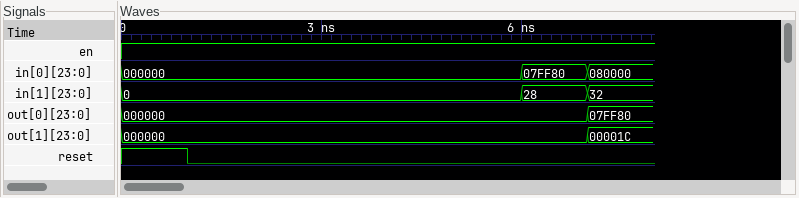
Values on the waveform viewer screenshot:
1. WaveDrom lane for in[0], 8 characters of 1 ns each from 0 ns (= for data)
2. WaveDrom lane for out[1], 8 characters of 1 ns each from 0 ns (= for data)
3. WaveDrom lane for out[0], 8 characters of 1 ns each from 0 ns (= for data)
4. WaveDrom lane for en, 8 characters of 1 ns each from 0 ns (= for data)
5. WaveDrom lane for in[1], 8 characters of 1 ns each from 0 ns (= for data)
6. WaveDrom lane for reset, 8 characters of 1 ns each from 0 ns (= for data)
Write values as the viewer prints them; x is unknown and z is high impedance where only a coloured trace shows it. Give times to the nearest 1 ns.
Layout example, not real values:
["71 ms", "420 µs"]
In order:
["{name: 'in[0]', wave: '=.....==', data: '000000 07FF80 080000'}", "{name: 'out[1]', wave: '=......=', data: '000000 00001C'}", "{name: 'out[0]', wave: '=......=', data: '000000 07FF80'}", "{name: 'en', wave: '1.......'}", "{name: 'in[1]', wave: '=.....==', data: '0 28 32'}", "{name: 'reset', wave: '10......'}"]
